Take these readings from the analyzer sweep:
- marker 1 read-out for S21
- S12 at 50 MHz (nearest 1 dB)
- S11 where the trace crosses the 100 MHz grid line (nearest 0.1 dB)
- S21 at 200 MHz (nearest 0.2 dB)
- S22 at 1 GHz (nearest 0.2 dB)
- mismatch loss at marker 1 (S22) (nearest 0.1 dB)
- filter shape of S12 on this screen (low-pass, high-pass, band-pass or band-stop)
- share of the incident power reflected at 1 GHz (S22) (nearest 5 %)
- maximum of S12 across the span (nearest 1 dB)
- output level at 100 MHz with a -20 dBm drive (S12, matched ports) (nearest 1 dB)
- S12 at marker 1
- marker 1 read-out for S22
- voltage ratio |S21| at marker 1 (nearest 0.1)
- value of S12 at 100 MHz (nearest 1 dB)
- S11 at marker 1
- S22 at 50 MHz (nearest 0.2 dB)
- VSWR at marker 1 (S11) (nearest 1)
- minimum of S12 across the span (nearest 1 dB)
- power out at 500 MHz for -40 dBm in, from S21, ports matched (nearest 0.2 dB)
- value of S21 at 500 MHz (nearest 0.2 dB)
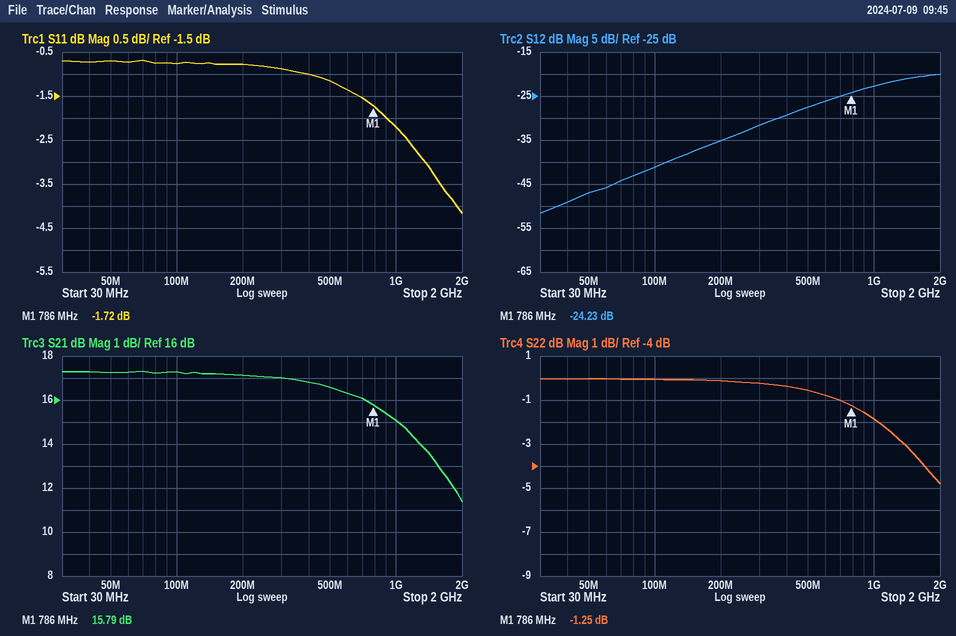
15.79 dB
-47 dB
-0.8 dB
17.2 dB
-1.8 dB
6.0 dB
high-pass
65 %
-20 dB
-61 dBm
-24.23 dB
-1.25 dB
6.2
-41 dB
-1.72 dB
0.0 dB
10
-52 dB
-23.4 dBm
16.6 dB
